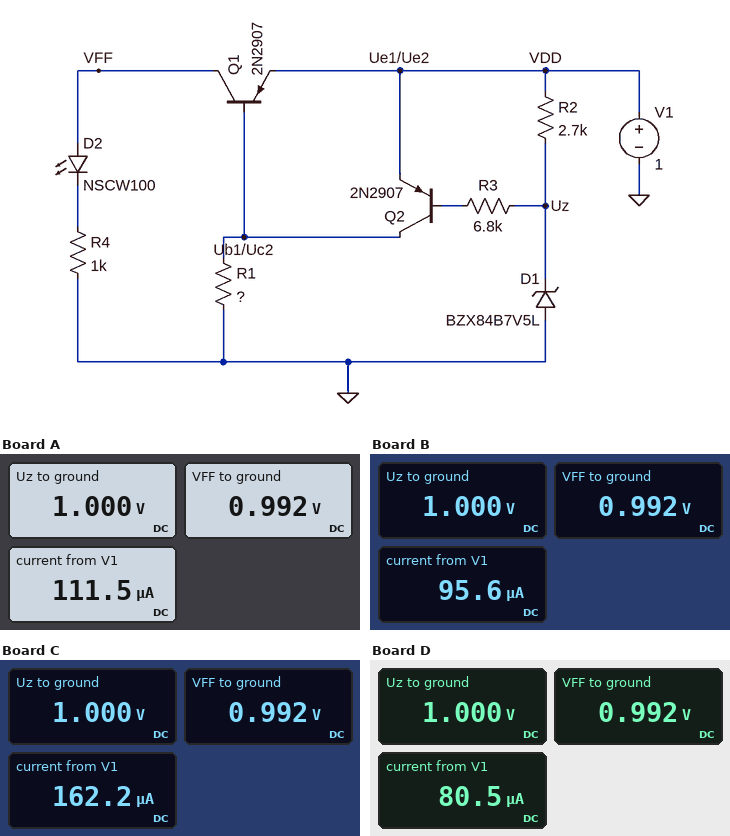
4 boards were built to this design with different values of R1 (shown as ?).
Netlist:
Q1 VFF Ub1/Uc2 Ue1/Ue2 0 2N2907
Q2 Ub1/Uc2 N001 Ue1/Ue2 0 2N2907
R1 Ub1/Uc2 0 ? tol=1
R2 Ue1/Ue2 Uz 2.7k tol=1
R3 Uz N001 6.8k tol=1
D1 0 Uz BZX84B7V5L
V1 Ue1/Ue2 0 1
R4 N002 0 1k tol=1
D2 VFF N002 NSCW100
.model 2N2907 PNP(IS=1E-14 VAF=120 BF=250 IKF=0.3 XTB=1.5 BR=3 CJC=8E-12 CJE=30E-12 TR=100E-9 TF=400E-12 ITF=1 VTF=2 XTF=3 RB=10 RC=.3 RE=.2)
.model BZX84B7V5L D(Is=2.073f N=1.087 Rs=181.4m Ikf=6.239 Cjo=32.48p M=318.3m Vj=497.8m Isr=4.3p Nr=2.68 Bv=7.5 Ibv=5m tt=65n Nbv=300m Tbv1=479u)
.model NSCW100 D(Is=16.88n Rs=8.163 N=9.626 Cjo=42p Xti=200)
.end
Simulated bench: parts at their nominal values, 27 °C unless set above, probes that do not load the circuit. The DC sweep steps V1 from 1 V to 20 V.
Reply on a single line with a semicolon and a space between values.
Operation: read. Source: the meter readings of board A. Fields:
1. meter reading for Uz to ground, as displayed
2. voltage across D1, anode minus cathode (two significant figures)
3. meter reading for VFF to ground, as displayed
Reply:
1.000 V; -1.0 V; 0.992 V
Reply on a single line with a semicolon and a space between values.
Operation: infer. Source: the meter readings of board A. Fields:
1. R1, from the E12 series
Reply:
3.3 kΩ
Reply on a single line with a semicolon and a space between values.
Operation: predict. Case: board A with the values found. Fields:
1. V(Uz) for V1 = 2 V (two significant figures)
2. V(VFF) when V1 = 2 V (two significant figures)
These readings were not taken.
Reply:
2.0 V; 2.0 V
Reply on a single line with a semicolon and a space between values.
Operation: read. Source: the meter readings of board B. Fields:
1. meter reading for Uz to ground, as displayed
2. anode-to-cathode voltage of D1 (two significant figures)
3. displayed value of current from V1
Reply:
1.000 V; -1.0 V; 95.6 µA
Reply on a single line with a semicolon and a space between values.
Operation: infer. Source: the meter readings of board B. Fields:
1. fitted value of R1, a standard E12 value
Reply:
3.9 kΩ
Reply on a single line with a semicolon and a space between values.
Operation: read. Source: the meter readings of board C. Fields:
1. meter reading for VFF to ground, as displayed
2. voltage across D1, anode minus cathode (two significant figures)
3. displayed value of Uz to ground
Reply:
0.992 V; -1.0 V; 1.000 V
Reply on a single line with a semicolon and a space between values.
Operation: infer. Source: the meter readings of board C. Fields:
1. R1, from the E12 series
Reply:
2.2 kΩ
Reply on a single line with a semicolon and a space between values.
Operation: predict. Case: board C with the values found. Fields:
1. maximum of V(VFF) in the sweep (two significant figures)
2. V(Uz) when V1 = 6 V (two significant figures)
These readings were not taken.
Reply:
8.2 V; 6.0 V
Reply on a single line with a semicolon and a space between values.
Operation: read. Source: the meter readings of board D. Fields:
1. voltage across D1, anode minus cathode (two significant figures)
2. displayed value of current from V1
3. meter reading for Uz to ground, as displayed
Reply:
-1.0 V; 80.5 µA; 1.000 V
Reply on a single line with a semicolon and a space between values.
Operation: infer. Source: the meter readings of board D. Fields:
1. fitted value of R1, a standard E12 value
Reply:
4.7 kΩ
